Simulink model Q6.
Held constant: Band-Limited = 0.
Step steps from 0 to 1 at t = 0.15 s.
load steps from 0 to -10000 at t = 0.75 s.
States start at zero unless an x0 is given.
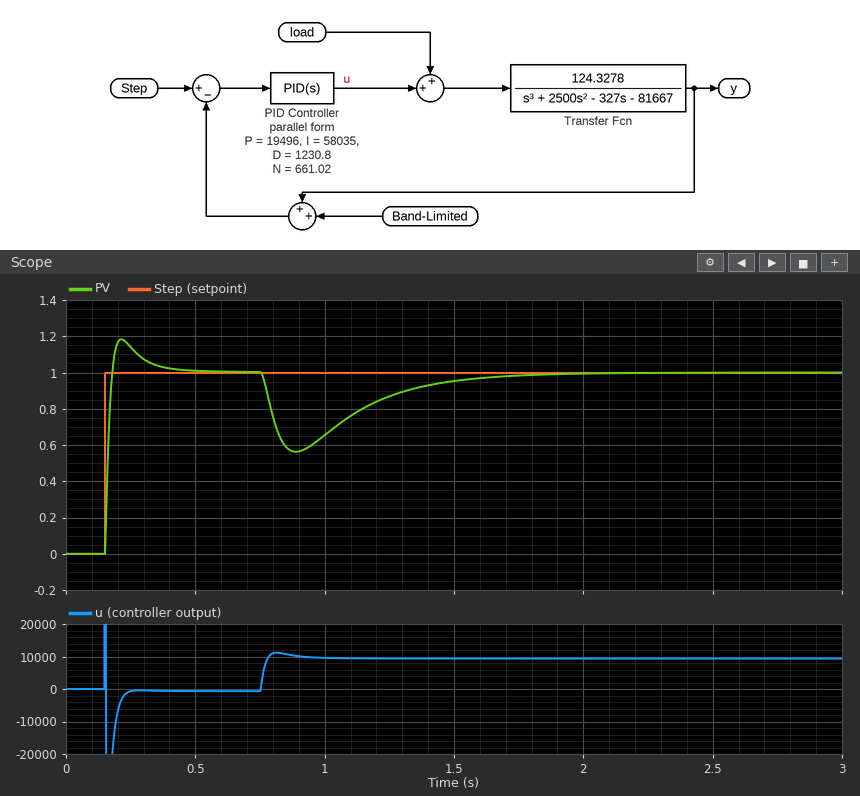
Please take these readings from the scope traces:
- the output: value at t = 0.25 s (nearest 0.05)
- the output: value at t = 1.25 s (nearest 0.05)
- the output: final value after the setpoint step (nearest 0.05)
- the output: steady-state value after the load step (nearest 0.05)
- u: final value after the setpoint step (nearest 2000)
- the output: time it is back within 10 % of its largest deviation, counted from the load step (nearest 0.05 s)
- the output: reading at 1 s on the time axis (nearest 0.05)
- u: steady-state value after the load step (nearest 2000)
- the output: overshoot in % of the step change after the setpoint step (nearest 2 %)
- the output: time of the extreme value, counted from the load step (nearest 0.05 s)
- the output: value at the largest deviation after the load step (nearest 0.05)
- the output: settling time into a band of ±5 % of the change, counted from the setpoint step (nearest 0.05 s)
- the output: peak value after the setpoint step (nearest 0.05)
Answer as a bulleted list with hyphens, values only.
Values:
- 1.15
- 0.85
- 1.00
- 1.00
- 0
- 0.75 s
- 0.65
- 10000
- 18 %
- 0.15 s
- 0.55
- 0.20 s
- 1.20
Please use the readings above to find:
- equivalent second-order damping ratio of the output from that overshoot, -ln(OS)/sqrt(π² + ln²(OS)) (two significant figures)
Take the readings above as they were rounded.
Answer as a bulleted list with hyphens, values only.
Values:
- 0.48
